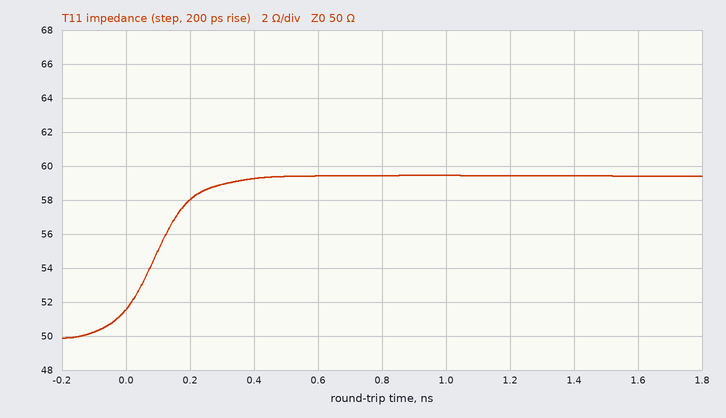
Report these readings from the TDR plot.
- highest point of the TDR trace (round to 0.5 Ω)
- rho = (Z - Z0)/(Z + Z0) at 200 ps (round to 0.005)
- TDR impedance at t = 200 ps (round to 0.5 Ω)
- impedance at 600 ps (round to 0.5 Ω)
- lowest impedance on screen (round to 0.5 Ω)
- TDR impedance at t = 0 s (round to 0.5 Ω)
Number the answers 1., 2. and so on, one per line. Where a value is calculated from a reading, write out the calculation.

1. 59.5 Ω
2. (58 − 50)/(58 + 50) ≈ +0.0741, so +0.075 to the nearest 0.005
3. 58.0 Ω
4. 59.5 Ω
5. 50.0 Ω
6. 51.5 Ω
